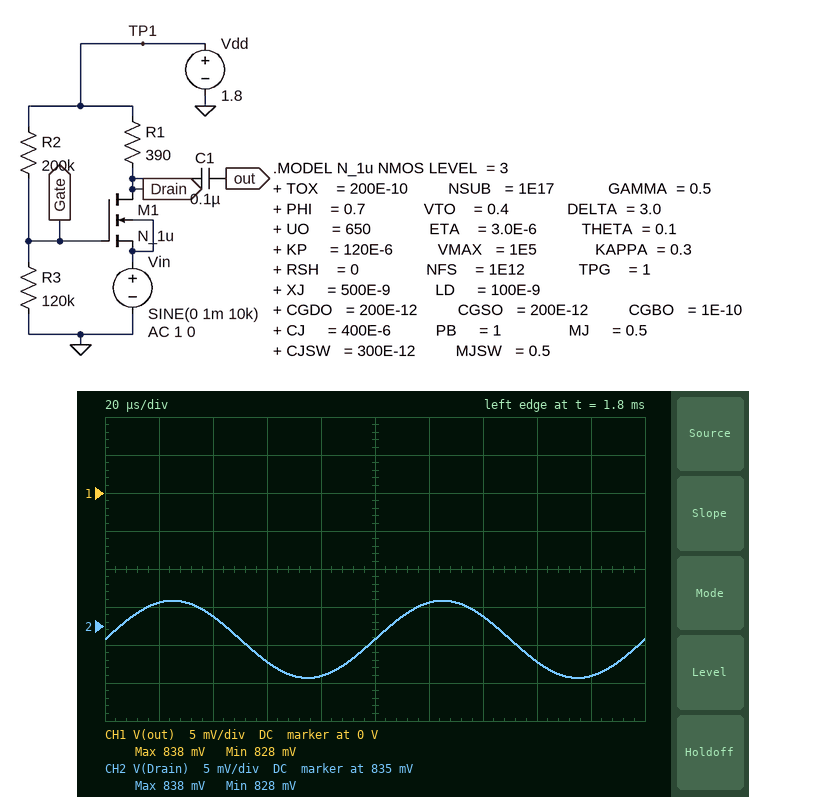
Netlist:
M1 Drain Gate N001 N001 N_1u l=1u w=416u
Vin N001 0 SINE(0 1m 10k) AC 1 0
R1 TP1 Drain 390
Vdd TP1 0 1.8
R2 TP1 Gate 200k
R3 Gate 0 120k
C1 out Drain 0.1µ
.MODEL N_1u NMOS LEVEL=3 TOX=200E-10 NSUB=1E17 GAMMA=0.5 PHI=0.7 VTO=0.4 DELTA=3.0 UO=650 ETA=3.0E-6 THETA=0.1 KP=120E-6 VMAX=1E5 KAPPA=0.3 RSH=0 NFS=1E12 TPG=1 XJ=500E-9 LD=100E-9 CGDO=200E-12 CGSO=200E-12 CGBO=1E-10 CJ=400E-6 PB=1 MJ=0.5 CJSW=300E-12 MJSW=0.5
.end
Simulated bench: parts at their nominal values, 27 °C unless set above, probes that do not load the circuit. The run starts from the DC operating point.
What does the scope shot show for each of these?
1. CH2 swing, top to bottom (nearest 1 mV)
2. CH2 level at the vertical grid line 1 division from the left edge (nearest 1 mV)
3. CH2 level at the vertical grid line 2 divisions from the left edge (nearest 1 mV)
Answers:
10 mV
838 mV
836 mV
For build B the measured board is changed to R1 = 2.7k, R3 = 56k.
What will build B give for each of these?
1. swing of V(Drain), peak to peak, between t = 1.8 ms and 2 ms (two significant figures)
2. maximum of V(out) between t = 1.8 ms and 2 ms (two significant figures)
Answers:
7.2 mV
1.6 V
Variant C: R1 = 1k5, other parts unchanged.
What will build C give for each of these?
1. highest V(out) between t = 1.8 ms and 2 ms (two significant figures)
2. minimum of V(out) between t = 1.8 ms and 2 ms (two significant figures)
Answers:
71 mV
68 mV
